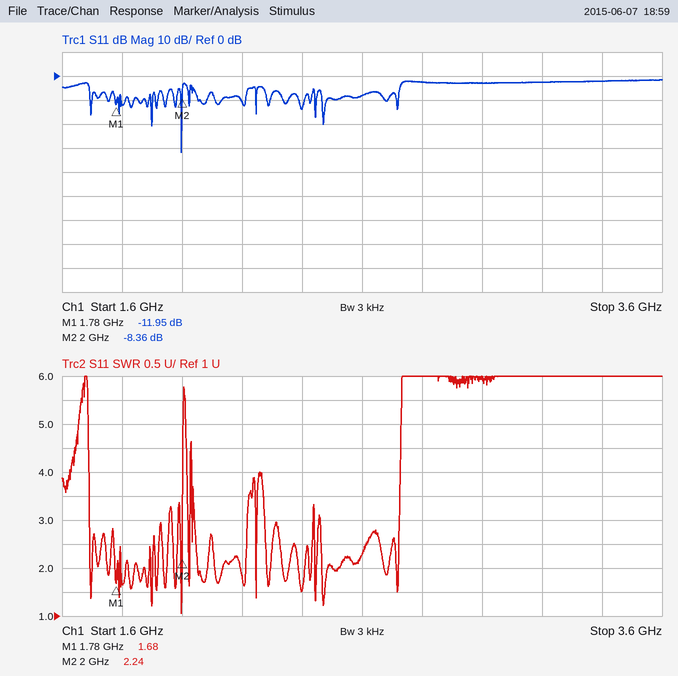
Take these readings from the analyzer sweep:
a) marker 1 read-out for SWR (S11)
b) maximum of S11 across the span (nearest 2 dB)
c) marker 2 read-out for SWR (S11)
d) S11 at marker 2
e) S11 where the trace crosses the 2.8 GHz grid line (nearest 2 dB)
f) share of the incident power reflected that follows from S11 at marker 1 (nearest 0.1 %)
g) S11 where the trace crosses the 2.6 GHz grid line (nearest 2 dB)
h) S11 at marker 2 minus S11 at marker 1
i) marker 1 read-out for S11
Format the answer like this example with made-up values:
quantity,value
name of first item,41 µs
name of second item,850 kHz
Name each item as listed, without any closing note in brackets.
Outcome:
quantity,value
marker 1 read-out for SWR,1.68
maximum of S11 across the span,-2 dB
marker 2 read-out for SWR,2.24
S11 at marker 2,-8.36 dB
S11 where the trace crosses the 2.8 GHz grid line,-2 dB
share of the incident power reflected that follows from S11 at marker 1,6.4 %
S11 where the trace crosses the 2.6 GHz grid line,-8 dB
S11 at marker 2 minus S11 at marker 1,3.59 dB
marker 1 read-out for S11,-11.95 dB
